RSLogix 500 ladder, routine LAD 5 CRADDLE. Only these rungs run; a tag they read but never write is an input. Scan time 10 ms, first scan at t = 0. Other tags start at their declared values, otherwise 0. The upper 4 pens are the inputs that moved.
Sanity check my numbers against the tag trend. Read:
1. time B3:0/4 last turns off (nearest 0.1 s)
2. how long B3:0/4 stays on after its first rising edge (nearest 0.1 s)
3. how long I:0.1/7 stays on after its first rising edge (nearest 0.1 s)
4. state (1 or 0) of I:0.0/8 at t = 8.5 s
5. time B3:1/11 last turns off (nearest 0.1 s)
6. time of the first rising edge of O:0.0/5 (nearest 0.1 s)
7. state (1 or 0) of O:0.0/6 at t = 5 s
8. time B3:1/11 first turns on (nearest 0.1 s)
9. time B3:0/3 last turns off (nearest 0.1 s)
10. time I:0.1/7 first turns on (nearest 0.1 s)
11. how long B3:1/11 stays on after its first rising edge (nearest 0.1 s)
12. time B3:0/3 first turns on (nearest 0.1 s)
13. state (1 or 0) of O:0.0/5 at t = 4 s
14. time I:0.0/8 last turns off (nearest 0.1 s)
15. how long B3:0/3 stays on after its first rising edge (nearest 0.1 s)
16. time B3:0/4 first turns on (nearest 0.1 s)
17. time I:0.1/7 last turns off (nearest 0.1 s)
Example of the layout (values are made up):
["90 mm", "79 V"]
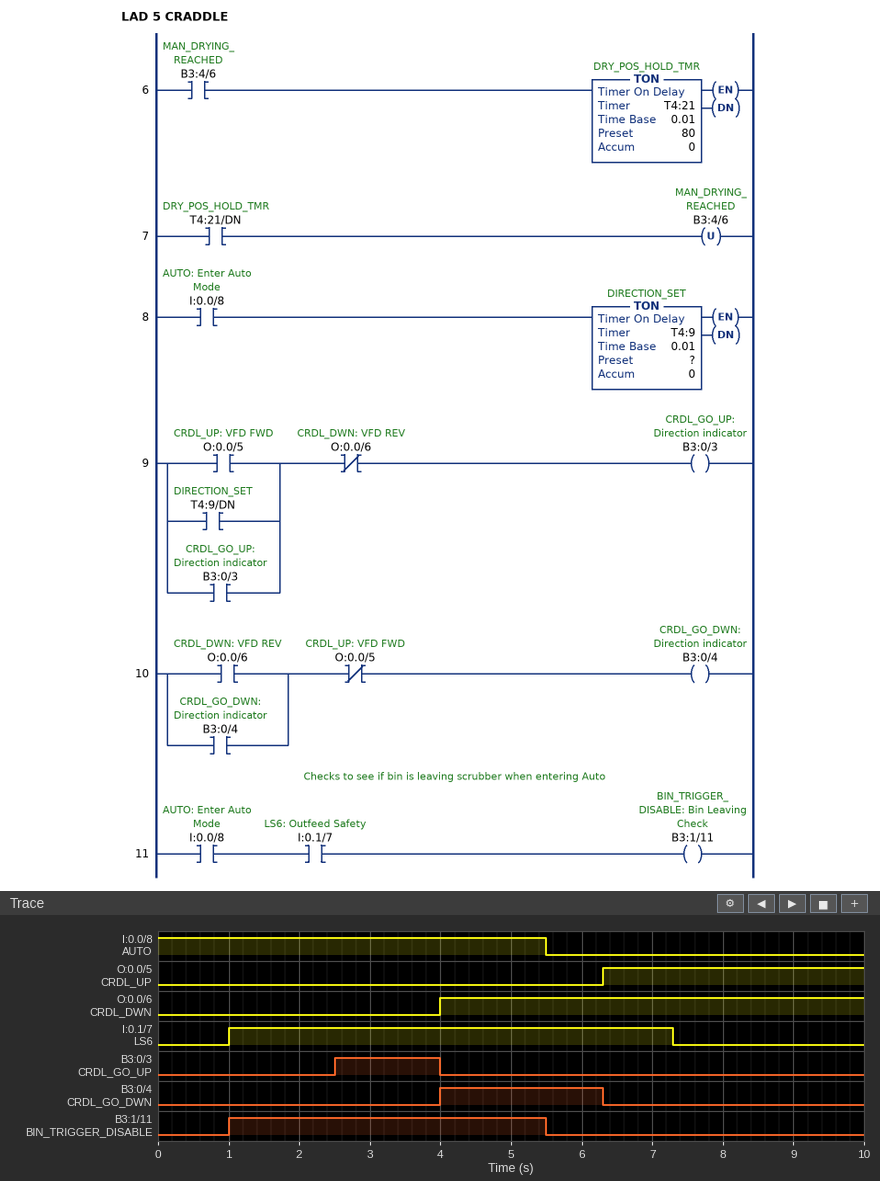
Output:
["6.3 s", "2.3 s", "6.3 s", "0", "5.5 s", "6.3 s", "1", "1.0 s", "4.0 s", "1.0 s", "4.5 s", "2.5 s", "0", "5.5 s", "1.5 s", "4.0 s", "7.3 s"]
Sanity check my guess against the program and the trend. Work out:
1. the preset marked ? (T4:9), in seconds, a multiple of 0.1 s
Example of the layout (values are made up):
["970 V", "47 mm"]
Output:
["2.5 s"]
